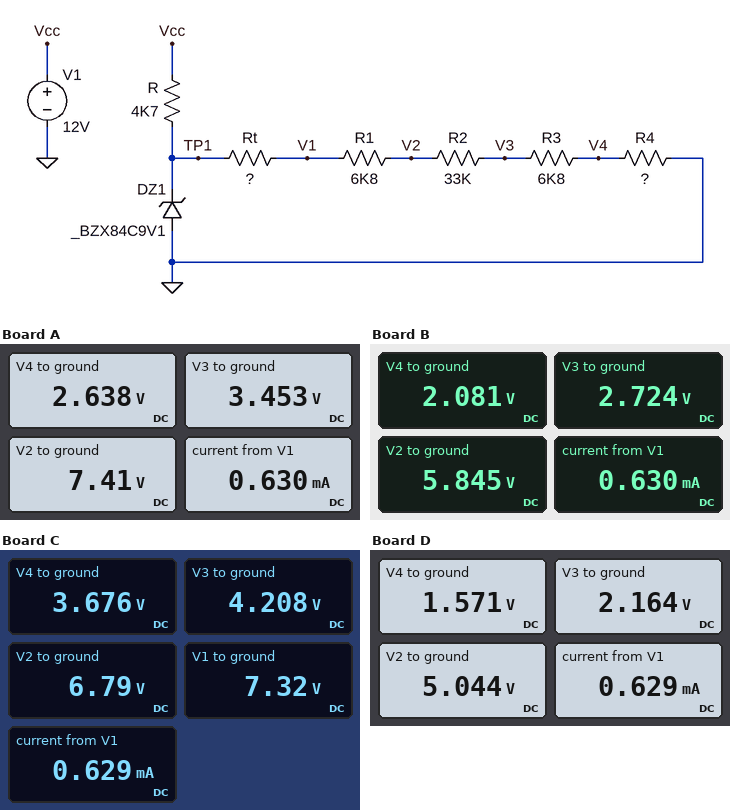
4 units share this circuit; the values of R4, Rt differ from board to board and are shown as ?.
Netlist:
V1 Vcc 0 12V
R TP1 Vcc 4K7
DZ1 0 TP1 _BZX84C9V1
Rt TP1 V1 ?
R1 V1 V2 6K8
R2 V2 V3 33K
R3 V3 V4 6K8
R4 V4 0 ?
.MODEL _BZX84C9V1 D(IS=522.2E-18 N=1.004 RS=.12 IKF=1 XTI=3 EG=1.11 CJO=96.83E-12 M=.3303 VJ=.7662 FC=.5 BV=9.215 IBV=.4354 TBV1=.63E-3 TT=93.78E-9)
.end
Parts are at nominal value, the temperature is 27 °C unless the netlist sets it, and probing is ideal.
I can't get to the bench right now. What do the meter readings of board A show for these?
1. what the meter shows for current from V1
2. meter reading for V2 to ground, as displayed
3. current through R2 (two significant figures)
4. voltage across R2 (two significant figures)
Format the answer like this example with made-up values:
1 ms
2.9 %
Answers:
0.630 mA
7.41 V
120 µA
4.0 V
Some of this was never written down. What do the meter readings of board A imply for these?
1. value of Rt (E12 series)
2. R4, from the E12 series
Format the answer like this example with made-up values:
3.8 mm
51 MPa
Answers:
6.8 kΩ
22 kΩ
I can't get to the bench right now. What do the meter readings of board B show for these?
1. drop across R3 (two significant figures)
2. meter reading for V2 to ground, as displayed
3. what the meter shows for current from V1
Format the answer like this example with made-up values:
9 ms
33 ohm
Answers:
640 mV
5.845 V
0.630 mA
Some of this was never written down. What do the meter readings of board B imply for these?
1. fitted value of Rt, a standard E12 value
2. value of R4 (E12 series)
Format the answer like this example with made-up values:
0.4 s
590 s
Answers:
27 kΩ
22 kΩ
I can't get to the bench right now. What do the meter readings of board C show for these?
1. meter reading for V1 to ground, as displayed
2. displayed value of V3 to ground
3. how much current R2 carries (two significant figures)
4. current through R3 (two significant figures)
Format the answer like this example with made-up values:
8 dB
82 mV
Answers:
7.32 V
4.208 V
78 µA
78 µA
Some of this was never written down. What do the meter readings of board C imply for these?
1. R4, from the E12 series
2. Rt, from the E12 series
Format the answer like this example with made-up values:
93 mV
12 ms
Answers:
47 kΩ
22 kΩ
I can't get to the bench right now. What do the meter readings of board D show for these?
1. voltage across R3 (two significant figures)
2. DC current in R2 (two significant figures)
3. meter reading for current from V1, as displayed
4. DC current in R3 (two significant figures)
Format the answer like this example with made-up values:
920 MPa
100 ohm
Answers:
590 mV
87 µA
0.629 mA
87 µA
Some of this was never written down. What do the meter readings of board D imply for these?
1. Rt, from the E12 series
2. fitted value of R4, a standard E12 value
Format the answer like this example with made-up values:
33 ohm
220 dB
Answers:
39 kΩ
18 kΩ
